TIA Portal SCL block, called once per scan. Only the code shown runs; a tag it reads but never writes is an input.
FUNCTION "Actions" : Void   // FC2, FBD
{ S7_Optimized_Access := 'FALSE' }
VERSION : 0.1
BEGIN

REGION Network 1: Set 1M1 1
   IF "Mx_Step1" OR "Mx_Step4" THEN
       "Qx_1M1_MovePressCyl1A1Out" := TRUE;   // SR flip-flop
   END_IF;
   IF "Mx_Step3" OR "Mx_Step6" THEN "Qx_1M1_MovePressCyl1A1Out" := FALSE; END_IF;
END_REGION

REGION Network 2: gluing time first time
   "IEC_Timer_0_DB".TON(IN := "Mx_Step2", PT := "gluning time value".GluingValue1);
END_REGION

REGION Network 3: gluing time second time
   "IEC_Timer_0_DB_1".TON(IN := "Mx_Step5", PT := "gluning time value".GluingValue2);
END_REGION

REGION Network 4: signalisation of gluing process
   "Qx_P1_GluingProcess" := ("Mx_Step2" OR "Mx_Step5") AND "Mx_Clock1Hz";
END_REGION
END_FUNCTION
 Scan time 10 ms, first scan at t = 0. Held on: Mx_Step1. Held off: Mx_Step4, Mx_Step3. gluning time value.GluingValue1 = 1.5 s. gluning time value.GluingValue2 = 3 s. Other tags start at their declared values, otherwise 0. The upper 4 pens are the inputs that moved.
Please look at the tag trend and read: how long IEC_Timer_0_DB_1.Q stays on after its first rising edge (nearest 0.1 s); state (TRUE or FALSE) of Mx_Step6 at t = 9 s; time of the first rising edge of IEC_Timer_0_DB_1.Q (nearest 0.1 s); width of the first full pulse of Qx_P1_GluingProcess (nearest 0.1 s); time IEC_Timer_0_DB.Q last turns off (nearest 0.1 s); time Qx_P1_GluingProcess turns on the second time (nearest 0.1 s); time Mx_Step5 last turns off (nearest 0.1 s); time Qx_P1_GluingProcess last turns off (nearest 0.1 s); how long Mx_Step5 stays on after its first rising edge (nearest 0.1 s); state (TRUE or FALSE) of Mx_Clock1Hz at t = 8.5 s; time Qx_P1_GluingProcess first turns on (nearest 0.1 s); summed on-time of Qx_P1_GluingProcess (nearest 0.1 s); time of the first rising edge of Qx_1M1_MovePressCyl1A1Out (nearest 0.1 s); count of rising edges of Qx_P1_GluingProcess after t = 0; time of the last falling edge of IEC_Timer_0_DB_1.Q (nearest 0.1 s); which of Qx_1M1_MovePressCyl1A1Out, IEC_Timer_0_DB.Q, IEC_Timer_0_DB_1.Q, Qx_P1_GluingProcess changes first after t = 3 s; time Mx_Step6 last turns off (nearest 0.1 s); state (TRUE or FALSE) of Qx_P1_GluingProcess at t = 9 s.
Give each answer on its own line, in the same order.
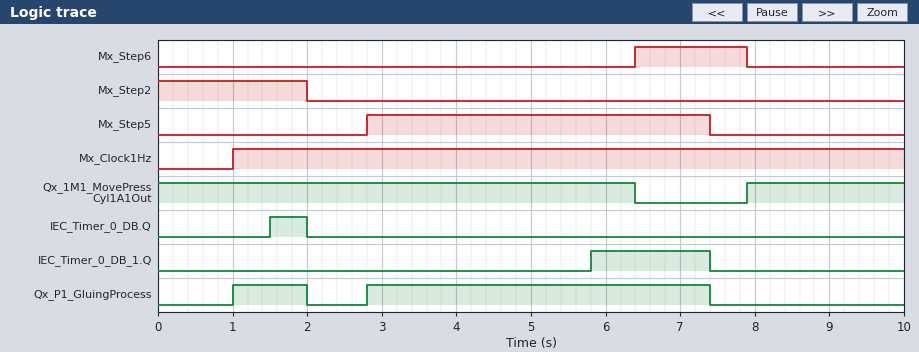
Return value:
1.6 s
FALSE
5.8 s
1.0 s
2.0 s
2.8 s
7.4 s
7.4 s
4.6 s
TRUE
1.0 s
5.6 s
7.9 s
2
7.4 s
IEC_Timer_0_DB_1.Q
7.9 s
FALSE
